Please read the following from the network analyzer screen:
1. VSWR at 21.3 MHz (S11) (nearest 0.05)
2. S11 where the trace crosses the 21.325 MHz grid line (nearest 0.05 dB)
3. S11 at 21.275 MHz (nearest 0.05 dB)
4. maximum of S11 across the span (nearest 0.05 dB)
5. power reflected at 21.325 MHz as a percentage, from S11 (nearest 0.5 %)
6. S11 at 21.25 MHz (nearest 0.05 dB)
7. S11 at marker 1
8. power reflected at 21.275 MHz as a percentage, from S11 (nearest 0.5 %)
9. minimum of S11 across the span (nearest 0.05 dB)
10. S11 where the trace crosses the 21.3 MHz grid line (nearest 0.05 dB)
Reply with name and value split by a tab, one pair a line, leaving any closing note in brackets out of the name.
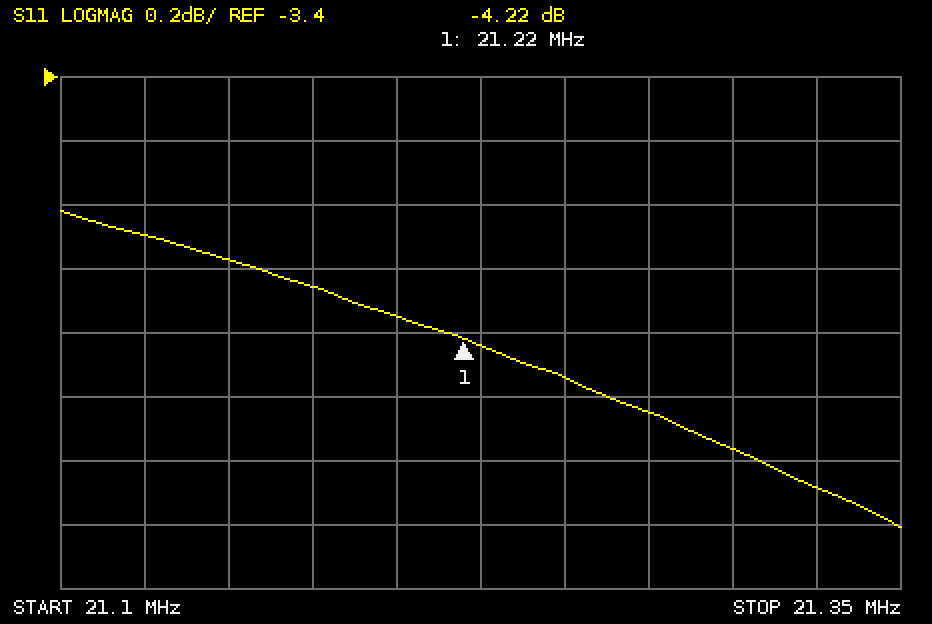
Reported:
VSWR at 21.3 MHz (S11)	3.90
S11 where the trace crosses the 21.325 MHz grid line	-4.70 dB
S11 at 21.275 MHz	-4.45 dB
maximum of S11 across the span	-3.80 dB
power reflected at 21.325 MHz as a percentage, from S11	34.0 %
S11 at 21.25 MHz	-4.35 dB
S11 at marker 1	-4.22 dB
power reflected at 21.275 MHz as a percentage, from S11	36.0 %
minimum of S11 across the span	-4.80 dB
S11 where the trace crosses the 21.3 MHz grid line	-4.55 dB
